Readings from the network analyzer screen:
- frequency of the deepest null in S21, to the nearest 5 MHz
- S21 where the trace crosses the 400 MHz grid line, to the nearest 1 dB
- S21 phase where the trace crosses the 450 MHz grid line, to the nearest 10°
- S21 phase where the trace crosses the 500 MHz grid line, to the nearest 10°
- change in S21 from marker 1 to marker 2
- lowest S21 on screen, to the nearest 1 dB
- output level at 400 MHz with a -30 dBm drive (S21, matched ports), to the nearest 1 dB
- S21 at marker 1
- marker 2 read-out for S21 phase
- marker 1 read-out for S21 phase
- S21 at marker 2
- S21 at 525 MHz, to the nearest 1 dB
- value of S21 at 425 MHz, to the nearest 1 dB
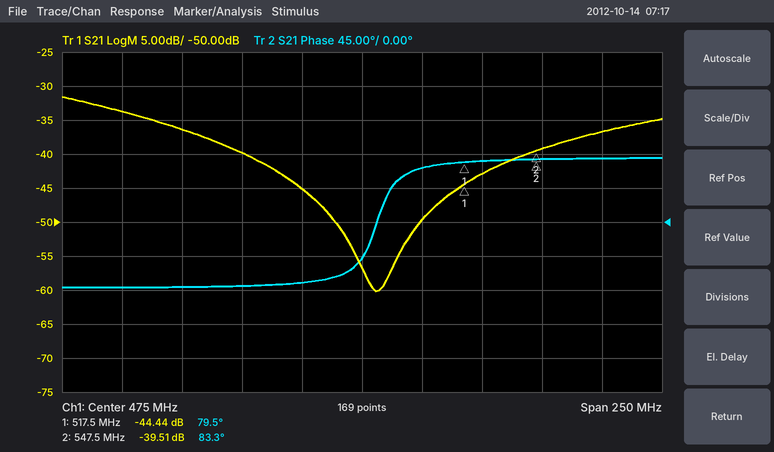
480 MHz
-36 dB
-80°
70°
4.93 dB
-60 dB
-66 dBm
-44.44 dB
83.3°
79.5°
-39.51 dB
-43 dB
-40 dB
